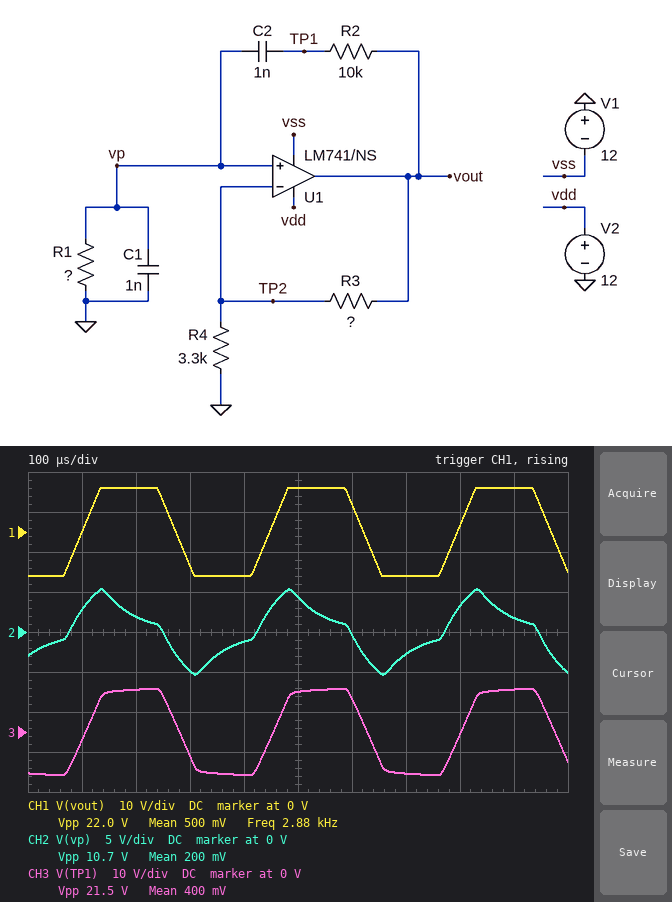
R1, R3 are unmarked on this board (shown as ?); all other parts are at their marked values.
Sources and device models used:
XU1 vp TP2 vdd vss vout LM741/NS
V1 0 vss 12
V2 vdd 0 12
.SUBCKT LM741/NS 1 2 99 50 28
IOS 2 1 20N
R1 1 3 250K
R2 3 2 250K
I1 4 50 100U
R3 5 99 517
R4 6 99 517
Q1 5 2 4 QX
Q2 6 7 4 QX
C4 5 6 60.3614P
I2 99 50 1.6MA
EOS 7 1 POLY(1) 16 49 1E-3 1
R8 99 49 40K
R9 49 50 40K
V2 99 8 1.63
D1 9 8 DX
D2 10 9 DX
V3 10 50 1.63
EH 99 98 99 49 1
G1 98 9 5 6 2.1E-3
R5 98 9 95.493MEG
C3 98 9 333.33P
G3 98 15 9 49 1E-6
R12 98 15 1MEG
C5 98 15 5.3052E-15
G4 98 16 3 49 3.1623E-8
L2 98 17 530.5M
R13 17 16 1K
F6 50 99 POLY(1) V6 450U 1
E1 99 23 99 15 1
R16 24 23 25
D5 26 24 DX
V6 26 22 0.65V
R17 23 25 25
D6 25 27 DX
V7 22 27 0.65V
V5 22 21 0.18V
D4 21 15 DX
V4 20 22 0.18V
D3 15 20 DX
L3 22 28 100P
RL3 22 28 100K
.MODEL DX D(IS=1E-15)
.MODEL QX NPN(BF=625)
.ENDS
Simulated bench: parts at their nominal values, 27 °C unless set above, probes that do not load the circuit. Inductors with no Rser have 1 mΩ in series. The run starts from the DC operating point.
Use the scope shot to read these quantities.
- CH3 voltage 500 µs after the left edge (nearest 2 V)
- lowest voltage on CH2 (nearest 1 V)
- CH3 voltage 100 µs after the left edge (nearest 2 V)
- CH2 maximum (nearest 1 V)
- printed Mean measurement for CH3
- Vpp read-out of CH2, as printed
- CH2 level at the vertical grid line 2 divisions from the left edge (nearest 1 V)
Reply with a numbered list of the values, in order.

1. 10 V
2. -5 V
3. -2 V
4. 5 V
5. 400 mV
6. 10.7 V
7. 2 V
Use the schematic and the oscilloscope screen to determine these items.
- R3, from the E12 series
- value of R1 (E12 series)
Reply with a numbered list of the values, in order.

1. 33 kΩ
2. 27 kΩ
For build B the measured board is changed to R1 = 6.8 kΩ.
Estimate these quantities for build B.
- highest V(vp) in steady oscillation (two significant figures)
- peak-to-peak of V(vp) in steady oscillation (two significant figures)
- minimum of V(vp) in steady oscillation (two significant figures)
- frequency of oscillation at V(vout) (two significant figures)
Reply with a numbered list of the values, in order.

1. 2.1 V
2. 4.1 V
3. -2.1 V
4. 5.7 kHz
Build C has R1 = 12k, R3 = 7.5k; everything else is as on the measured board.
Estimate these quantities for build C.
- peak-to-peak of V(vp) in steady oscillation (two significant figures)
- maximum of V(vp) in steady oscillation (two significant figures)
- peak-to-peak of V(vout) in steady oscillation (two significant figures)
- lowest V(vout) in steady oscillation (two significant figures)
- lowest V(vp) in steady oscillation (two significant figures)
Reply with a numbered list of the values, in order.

1. 5.4 V
2. 2.7 V
3. 18 V
4. -8.8 V
5. -2.7 V
